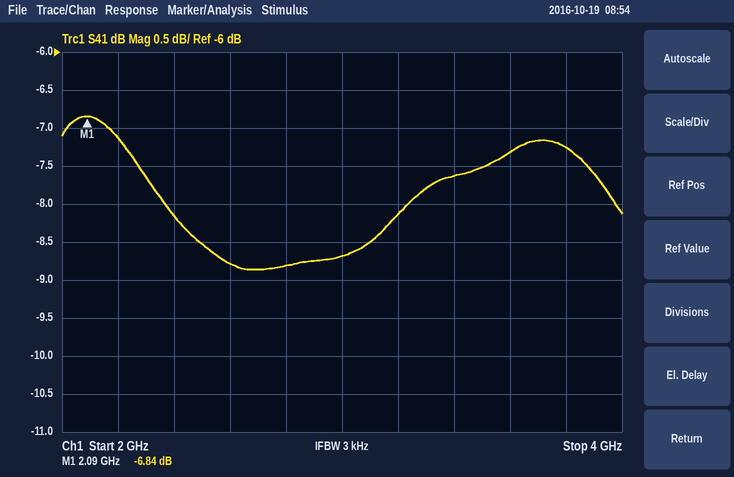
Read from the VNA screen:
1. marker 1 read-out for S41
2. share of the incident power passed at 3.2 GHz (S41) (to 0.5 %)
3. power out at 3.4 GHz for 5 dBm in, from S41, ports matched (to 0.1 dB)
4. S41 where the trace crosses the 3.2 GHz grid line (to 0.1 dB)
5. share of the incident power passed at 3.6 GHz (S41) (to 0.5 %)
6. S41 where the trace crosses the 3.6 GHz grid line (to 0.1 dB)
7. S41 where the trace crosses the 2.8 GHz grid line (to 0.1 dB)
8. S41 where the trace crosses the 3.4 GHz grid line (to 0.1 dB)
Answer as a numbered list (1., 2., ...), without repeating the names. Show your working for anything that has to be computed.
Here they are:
1. -6.84 dB
2. 10^(-8.1/10) ≈ 15.5 %
3. 5 dBm + (-7.6 dB) = -2.6 dBm
4. -8.1 dB
5. 10^(-7.3/10) ≈ 18.6 %, so 18.5 % to the nearest 0.5 %
6. -7.3 dB
7. -8.8 dB
8. -7.6 dB
